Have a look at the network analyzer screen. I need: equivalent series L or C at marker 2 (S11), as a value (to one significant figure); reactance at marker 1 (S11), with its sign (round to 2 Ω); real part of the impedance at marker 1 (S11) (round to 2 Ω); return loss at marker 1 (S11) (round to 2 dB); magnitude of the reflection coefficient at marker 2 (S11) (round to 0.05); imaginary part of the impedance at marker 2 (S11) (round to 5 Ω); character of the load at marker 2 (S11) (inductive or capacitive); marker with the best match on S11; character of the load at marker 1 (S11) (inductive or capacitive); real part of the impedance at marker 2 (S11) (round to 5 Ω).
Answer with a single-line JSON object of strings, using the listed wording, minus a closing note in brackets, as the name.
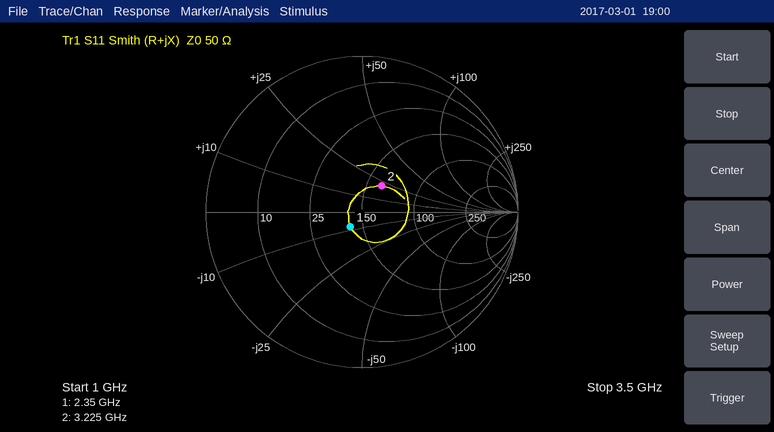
{"equivalent series L or C at marker 2 (S11), as a value": "1 nH", "reactance at marker 1 (S11), with its sign": "-8 Ω", "real part of the impedance at marker 1 (S11)": "42 Ω", "return loss at marker 1 (S11)": "18 dB", "magnitude of the reflection coefficient at marker 2 (S11)": "0.20", "imaginary part of the impedance at marker 2 (S11)": "+20 Ω", "character of the load at marker 2 (S11)": "inductive", "marker with the best match on S11": "marker 1", "character of the load at marker 1 (S11)": "capacitive", "real part of the impedance at marker 2 (S11)": "60 Ω"}
